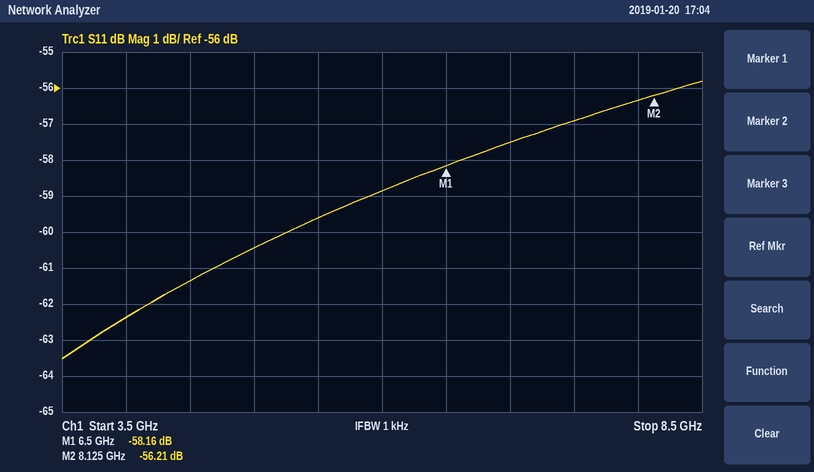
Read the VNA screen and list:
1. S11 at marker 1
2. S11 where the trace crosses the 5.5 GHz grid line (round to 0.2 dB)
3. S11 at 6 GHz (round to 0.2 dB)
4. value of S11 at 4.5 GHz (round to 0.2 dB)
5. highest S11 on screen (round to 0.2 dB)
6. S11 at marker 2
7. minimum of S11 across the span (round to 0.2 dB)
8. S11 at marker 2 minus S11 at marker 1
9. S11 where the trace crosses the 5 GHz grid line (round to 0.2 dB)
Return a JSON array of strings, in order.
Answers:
["-58.16 dB", "-59.6 dB", "-58.8 dB", "-61.4 dB", "-55.8 dB", "-56.21 dB", "-63.6 dB", "1.95 dB", "-60.4 dB"]
